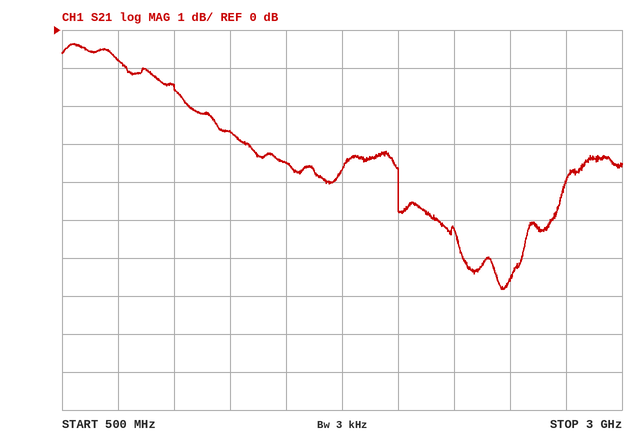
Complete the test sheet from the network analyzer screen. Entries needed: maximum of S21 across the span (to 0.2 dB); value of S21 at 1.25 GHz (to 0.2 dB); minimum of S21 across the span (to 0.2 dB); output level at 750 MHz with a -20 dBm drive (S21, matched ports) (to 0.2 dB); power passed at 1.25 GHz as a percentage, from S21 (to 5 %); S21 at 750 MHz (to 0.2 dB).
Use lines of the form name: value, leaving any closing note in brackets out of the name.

maximum of S21 across the span: -0.4 dB
value of S21 at 1.25 GHz: -2.6 dB
minimum of S21 across the span: -6.8 dB
output level at 750 MHz with a -20 dBm drive (S21, matched ports): -20.8 dBm
power passed at 1.25 GHz as a percentage, from S21: 55 %
S21 at 750 MHz: -0.8 dB
